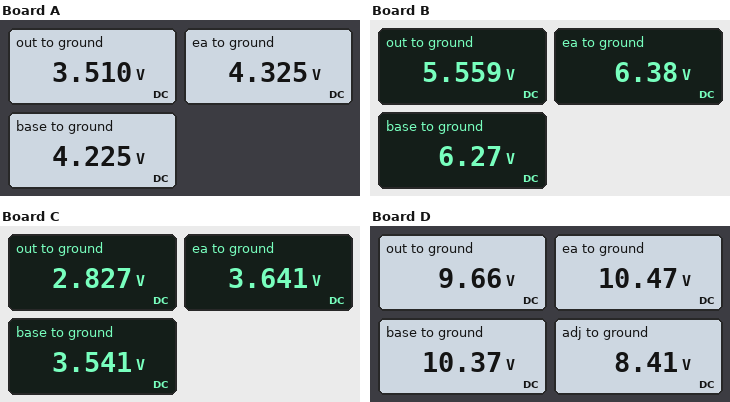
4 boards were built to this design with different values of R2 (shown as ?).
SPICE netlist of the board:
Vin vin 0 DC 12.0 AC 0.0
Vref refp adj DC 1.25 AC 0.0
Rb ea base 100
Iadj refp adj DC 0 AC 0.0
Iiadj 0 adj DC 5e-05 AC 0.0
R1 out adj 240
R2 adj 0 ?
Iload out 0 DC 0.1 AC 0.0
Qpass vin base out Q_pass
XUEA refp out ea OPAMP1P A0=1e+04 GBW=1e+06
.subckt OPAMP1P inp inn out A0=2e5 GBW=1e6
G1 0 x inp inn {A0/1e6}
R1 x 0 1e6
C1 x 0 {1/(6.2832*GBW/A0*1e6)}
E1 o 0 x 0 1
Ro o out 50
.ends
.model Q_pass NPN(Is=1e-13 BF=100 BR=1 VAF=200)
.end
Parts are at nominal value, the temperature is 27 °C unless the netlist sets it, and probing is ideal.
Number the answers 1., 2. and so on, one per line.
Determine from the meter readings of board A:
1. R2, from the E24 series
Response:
1. 430 Ω
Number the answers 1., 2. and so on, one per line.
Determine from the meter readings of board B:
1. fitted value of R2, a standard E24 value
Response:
1. 820 Ω
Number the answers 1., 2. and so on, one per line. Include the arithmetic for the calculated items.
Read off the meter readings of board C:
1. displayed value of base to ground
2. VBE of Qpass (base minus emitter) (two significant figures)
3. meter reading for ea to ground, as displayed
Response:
1. 3.541 V
2. 3.541 V - 2.827 V = 710 mV
3. 3.641 V
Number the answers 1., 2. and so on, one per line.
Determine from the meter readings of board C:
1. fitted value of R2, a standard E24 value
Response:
1. 300 Ω
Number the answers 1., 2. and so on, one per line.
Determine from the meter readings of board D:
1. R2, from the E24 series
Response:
1. 1.6 kΩ
